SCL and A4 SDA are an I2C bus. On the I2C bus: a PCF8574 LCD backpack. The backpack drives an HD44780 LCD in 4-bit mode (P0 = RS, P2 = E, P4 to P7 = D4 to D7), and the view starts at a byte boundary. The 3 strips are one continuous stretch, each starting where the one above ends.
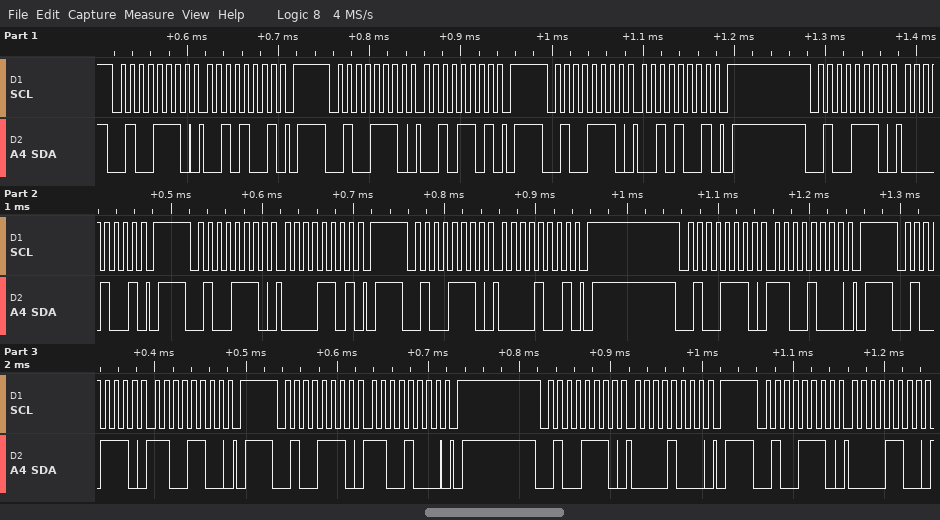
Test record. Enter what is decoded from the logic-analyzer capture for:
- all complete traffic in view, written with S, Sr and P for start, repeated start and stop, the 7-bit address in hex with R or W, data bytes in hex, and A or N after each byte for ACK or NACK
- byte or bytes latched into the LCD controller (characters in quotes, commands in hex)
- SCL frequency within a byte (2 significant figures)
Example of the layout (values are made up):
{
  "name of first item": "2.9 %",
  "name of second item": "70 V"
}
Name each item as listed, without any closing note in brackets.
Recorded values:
{
  "all complete traffic in view, written with S, Sr and P for start, repeated start and stop, the 7-bit address in hex with R or W, data bytes in hex, and A or N after each byte for ACK or NACK": "S 27W A 29 A P S 27W A 2D A P S 27W A 29 A P S 27W A 09 A P S 27W A 0D A P S 27W A 09 A P S 27W A C8 A P S 27W A CC A P S 27W A C8 A P S 27W A 08 A P S 27W A 0C A",
  "byte or bytes latched into the LCD controller": "' '",
  "SCL frequency within a byte": "100 kHz"
}
